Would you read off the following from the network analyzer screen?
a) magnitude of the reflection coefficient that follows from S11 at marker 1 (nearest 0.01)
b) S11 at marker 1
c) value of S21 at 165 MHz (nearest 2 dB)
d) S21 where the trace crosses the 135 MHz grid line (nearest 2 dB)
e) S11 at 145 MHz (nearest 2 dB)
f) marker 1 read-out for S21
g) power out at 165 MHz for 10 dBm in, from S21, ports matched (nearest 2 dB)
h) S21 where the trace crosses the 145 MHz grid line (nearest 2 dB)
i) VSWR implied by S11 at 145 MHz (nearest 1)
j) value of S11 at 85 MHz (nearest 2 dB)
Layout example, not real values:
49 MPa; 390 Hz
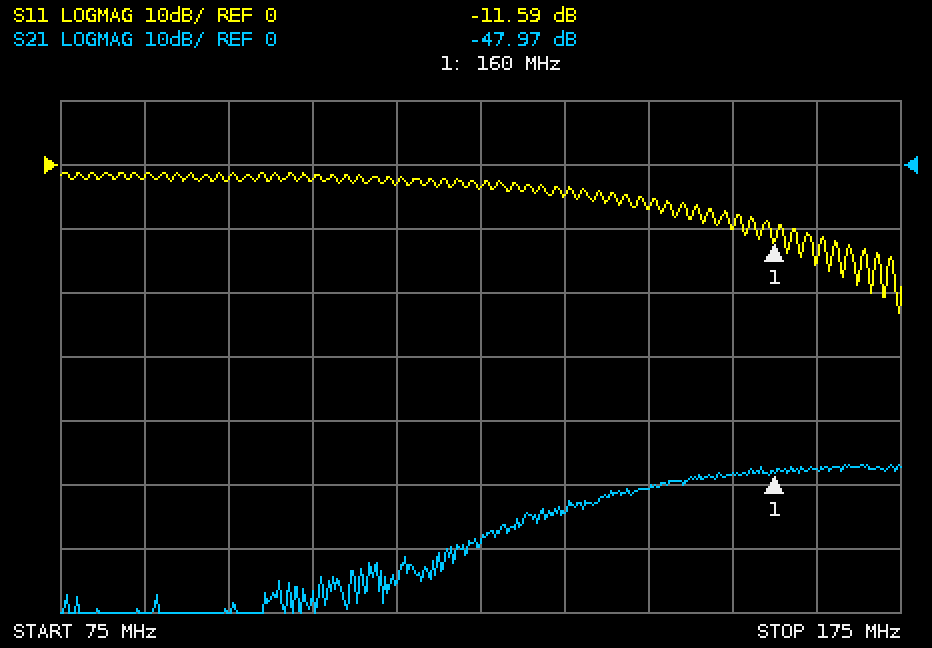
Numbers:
0.26; -11.59 dB; -48 dB; -54 dB; -6 dB; -47.97 dB; -38 dBm; -50 dB; 3; -2 dB
